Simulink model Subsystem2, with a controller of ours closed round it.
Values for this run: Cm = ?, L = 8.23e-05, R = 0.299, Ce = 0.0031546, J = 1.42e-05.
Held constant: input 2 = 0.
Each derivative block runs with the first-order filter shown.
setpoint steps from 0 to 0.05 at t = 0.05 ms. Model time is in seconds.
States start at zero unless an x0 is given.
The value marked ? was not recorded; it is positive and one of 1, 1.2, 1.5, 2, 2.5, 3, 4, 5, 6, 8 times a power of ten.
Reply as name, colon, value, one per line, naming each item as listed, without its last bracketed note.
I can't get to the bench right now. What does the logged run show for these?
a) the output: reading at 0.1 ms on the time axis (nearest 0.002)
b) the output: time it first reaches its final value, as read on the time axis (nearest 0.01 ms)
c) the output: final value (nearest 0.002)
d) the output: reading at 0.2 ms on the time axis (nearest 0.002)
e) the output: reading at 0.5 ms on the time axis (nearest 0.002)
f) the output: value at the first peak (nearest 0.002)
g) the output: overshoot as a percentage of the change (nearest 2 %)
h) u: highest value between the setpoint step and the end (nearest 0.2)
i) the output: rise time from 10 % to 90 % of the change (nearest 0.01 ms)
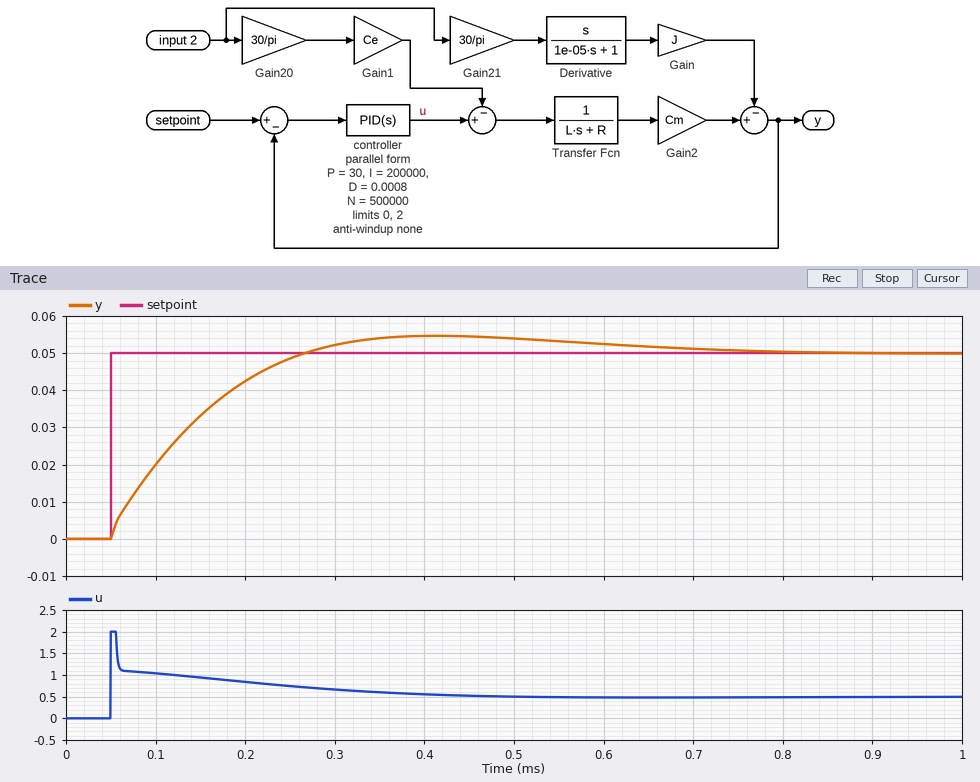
the output: reading at 0.1 ms on the time axis: 0.020
the output: time it first reaches its final value, as read on the time axis: 0.27 ms
the output: final value: 0.050
the output: reading at 0.2 ms on the time axis: 0.042
the output: reading at 0.5 ms on the time axis: 0.054
the output: value at the first peak: 0.054
the output: overshoot as a percentage of the change: 10 %
u: highest value between the setpoint step and the end: 2.0
the output: rise time from 10 % to 90 % of the change: 0.16 ms
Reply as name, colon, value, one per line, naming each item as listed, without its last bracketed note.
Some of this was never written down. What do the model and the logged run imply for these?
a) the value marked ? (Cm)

the value marked ?: 0.03
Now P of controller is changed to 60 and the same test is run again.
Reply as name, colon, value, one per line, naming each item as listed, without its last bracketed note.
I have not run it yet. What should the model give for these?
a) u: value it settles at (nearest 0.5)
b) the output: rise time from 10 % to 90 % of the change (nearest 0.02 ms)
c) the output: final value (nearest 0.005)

u: value it settles at: 0.5
the output: rise time from 10 % to 90 % of the change: 0.12 ms
the output: final value: 0.050
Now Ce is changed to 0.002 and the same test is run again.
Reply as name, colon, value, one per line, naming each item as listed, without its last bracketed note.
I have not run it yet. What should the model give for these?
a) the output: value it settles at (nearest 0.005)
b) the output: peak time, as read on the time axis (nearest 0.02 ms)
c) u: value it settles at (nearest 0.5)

the output: value it settles at: 0.050
the output: peak time, as read on the time axis: 0.42 ms
u: value it settles at: 0.5
